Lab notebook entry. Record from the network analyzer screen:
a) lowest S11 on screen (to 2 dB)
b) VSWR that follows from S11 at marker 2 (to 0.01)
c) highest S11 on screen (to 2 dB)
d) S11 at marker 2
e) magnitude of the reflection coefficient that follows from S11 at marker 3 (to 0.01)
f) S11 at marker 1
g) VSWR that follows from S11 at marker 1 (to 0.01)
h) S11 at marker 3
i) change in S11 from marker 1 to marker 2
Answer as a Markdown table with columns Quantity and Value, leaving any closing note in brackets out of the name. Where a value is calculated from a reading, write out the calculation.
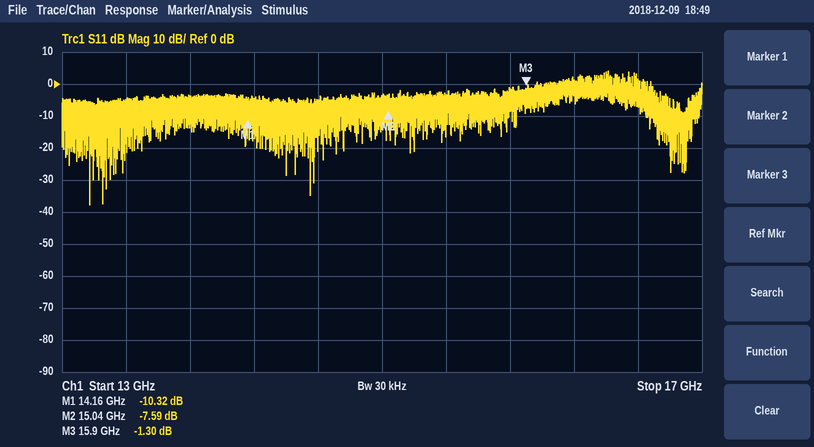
| Quantity | Value |
|---|---|
| lowest S11 on screen | -38 dB |
| VSWR that follows from S11 at marker 2 | (1 + 0.4173)/(1 − 0.4173) ≈ 2.43 |
| highest S11 on screen | 4 dB |
| S11 at marker 2 | -7.59 dB |
| magnitude of the reflection coefficient that follows from S11 at marker 3 | 10^(-1.3/20) ≈ 0.86 |
| S11 at marker 1 | -10.32 dB |
| VSWR that follows from S11 at marker 1 | (1 + 0.3048)/(1 − 0.3048) ≈ 1.88 |
| S11 at marker 3 | -1.30 dB |
| change in S11 from marker 1 to marker 2 | -7.59 − (-10.32) = 2.73 dB |
